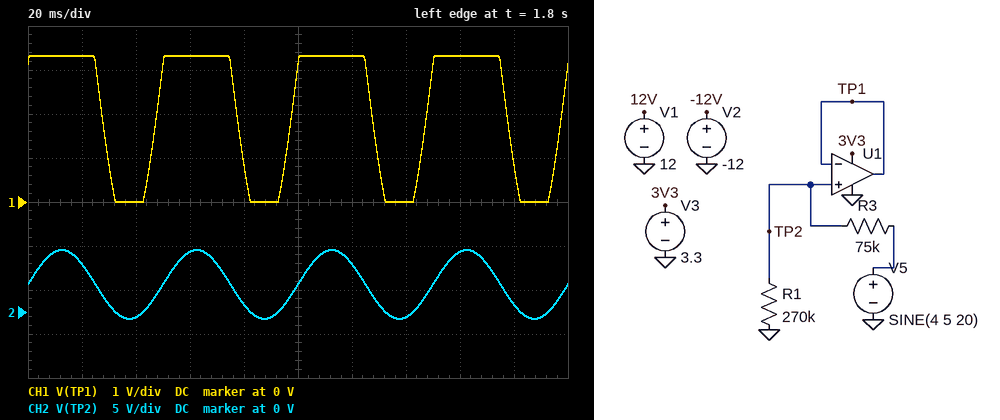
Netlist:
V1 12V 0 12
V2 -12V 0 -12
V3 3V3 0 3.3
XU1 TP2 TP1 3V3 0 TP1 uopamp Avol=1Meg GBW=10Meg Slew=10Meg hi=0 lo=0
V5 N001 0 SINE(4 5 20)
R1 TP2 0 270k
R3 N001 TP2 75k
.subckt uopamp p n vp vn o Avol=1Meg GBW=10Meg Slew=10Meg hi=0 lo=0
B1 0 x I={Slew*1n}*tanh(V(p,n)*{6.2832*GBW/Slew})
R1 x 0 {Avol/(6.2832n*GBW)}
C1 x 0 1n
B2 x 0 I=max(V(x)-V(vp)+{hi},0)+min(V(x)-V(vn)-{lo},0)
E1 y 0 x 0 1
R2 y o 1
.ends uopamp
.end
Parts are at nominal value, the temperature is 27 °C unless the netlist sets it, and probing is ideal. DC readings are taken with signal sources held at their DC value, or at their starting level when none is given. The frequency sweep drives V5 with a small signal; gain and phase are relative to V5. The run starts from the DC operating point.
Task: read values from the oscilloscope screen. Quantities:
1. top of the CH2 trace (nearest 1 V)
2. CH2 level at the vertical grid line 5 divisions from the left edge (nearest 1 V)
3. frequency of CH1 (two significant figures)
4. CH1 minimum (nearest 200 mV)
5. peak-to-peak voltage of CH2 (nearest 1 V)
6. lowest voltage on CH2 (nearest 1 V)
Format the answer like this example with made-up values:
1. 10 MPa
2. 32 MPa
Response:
1. 7 V
2. 3 V
3. 20 Hz
4. 0 V
5. 8 V
6. -1 V
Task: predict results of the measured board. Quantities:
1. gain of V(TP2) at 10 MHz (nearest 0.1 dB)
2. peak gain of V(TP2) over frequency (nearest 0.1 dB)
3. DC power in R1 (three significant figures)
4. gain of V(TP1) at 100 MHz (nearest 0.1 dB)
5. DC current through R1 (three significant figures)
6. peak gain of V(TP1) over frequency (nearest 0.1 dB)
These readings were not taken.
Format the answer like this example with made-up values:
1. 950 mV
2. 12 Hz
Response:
1. -2.1 dB
2. -2.1 dB
3. 36.3 µW
4. -22.2 dB
5. 11.6 µA
6. -2.1 dB
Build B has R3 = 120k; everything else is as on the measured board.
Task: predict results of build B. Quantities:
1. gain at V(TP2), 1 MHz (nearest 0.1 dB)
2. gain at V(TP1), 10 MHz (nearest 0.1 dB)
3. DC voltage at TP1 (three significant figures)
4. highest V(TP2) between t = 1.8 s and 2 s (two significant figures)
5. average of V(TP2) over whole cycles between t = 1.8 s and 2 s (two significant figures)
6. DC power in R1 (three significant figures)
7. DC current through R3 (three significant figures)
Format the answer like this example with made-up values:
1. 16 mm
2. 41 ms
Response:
1. -3.2 dB
2. -6.2 dB
3. 2.77 V
4. 6.2 V
5. 2.8 V
6. 28.4 µW
7. 10.3 µA
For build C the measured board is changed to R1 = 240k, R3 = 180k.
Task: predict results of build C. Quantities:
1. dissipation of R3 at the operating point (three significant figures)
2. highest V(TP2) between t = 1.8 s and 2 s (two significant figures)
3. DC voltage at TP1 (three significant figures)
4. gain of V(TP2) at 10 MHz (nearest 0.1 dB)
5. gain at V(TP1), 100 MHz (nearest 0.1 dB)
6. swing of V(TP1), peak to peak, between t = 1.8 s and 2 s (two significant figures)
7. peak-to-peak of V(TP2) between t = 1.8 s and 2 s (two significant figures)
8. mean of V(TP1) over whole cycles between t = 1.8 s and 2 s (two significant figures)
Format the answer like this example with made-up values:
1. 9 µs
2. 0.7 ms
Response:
1. 16.3 µW
2. 5.1 V
3. 2.29 V
4. -4.9 dB
5. -24.9 dB
6. 3.3 V
7. 5.7 V
8. 1.9 V
